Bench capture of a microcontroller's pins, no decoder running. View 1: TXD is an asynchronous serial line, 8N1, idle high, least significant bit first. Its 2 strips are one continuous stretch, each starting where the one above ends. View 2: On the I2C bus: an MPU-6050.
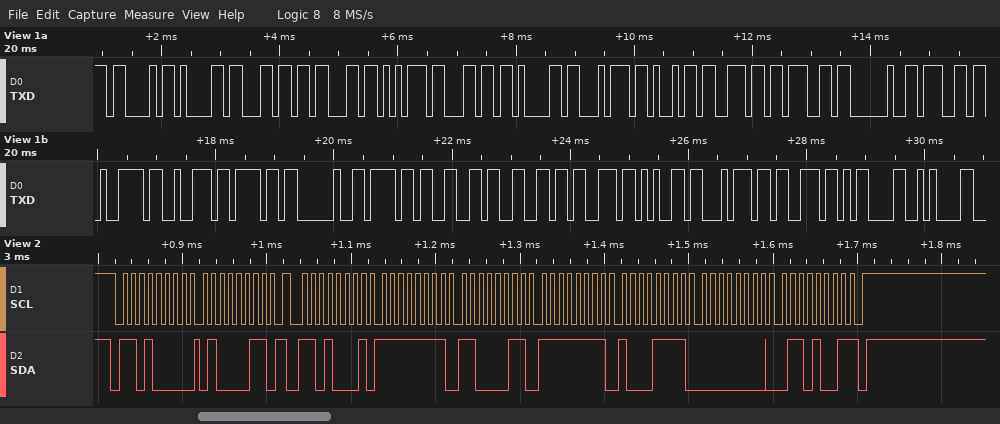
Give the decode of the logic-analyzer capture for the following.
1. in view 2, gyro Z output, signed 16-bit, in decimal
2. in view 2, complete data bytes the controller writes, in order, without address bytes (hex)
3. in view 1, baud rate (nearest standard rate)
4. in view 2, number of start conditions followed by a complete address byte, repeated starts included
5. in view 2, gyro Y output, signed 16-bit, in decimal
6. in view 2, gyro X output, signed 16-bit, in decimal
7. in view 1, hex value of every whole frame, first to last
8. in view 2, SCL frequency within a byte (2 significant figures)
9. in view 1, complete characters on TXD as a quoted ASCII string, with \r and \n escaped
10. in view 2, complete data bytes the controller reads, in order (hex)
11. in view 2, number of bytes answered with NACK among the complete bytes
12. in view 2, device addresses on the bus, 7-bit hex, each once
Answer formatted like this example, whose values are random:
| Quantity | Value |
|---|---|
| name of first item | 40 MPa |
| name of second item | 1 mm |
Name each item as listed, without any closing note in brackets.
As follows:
| Quantity | Value |
|---|---|
| in view 2, gyro Z output, signed 16-bit, in decimal | 105 |
| in view 2, complete data bytes the controller writes, in order, without address bytes | 43 |
| in view 1, baud rate | 9600 baud |
| in view 2, number of start conditions followed by a complete address byte, repeated starts included | 2 |
| in view 2, gyro Y output, signed 16-bit, in decimal | -113 |
| in view 2, gyro X output, signed 16-bit, in decimal | -61 |
| in view 1, hex value of every whole frame, first to last | 0x43 0x61 0x6C 0x63 0x75 0x6C 0x61 0x74 0x69 0x6E 0x67 0x20 0x67 0x79 0x72 0x6F 0x20 0x6F 0x66 0x66 0x73 0x65 0x74 0x73 0x0D 0x0A |
| in view 2, SCL frequency within a byte | 100 kHz |
| in view 1, complete characters on TXD as a quoted ASCII string, with \r and \n escaped | "Calculating gyro offsets\r\n" |
| in view 2, complete data bytes the controller reads, in order | FF C3 FF 8F 00 69 |
| in view 2, number of bytes answered with NACK among the complete bytes | 1 |
| in view 2, device addresses on the bus, 7-bit hex, each once | 0x68 |
